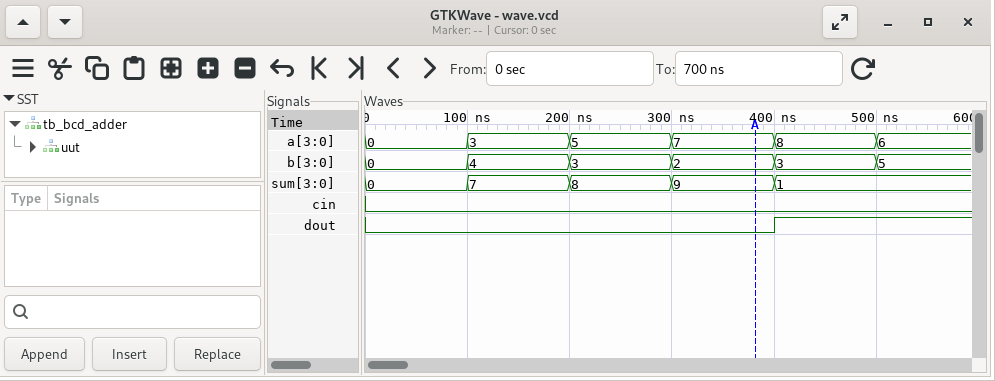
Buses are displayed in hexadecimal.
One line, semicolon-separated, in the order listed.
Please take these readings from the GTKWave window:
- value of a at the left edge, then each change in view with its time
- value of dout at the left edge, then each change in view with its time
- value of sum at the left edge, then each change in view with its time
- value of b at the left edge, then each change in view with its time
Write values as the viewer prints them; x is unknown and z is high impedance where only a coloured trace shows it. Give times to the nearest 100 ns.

0, 3 at 100 ns, 5 at 200 ns, 7 at 300 ns, 8 at 400 ns, 6 at 500 ns; 0, 1 at 400 ns; 0, 7 at 100 ns, 8 at 200 ns, 9 at 300 ns, 1 at 400 ns; 0, 4 at 100 ns, 3 at 200 ns, 2 at 300 ns, 3 at 400 ns, 5 at 500 ns
